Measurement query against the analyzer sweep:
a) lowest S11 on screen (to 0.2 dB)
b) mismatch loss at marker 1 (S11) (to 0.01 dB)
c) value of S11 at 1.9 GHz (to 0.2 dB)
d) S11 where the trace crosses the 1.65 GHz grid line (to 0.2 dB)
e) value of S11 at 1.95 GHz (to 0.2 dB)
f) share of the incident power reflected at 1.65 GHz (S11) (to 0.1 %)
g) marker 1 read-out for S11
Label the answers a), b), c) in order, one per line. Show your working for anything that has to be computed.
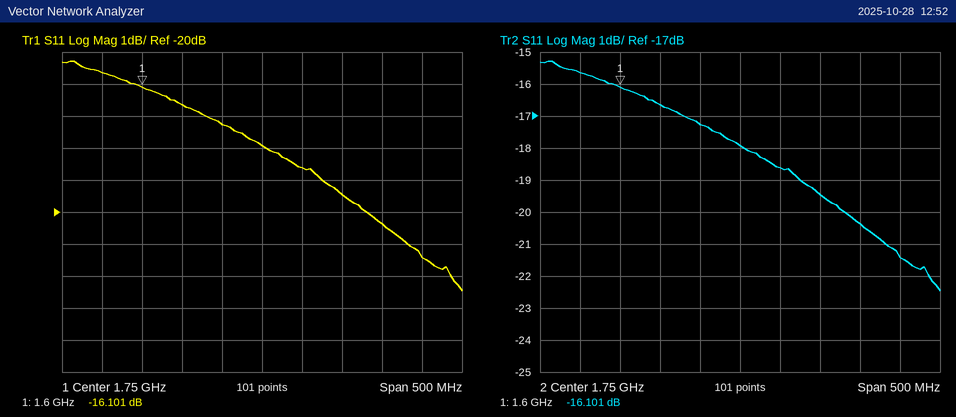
a) -22.4 dB
b) −10 log10(1 − 10^(-16.101/10)) ≈ 0.11 dB
c) -20.4 dB
d) -16.6 dB
e) -21.4 dB
f) 10^(-16.6/10) ≈ 2.2 %
g) -16.101 dB
